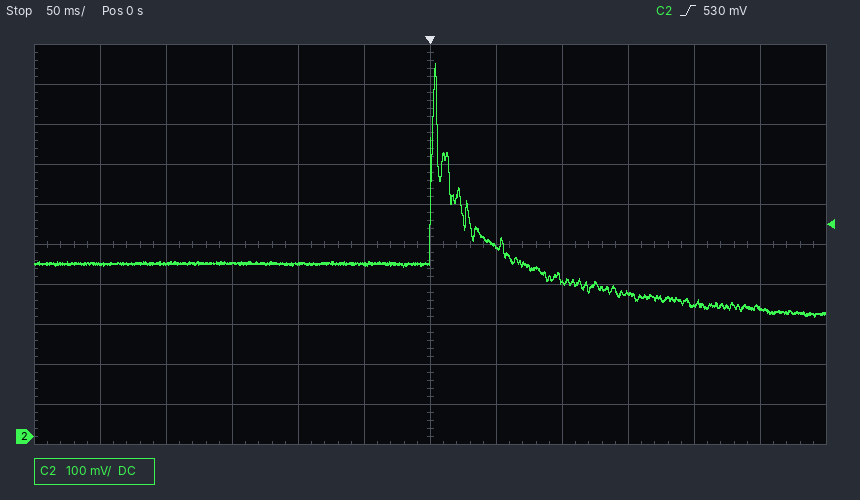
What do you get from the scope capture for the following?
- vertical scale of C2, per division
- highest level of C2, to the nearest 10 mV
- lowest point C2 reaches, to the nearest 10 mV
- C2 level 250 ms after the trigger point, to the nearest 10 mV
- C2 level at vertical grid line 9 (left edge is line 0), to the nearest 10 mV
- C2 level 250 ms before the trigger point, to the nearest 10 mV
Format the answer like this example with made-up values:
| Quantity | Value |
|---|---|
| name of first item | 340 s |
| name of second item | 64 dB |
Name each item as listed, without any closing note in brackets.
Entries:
| Quantity | Value |
|---|---|
| vertical scale of C2, per division | 100 mV |
| highest level of C2, to the nearest 10 mV | 930 mV |
| lowest point C2 reaches, to the nearest 10 mV | 300 mV |
| C2 level 250 ms after the trigger point, to the nearest 10 mV | 320 mV |
| C2 level at vertical grid line 9 (left edge is line 0), to the nearest 10 mV | 360 mV |
| C2 level 250 ms before the trigger point, to the nearest 10 mV | 430 mV |
